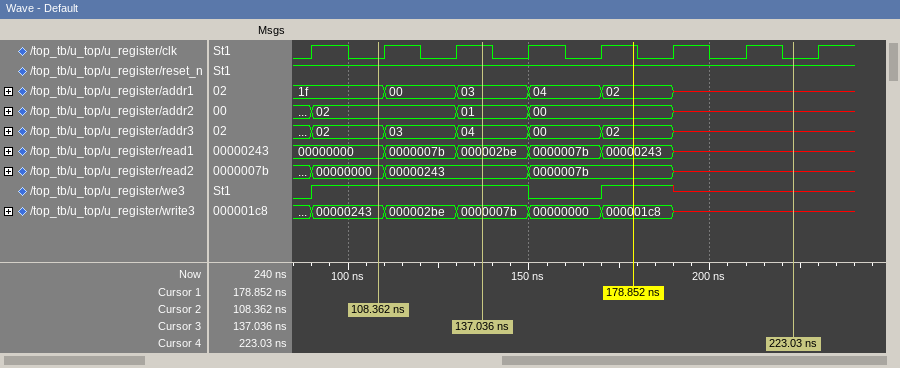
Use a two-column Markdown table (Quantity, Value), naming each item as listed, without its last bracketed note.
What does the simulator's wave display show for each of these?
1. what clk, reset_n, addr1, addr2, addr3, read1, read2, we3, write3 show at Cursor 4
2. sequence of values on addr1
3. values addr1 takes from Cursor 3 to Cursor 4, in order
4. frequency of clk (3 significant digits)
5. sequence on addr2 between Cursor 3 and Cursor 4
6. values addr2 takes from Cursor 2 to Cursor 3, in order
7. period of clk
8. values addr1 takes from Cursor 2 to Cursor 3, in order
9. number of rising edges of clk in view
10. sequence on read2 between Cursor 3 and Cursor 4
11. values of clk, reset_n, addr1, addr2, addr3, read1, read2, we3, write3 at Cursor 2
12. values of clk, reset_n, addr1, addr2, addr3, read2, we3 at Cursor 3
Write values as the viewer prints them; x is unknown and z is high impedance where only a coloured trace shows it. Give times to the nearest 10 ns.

| Quantity | Value |
|---|---|
| what clk, reset_n, addr1, addr2, addr3, read1, read2, we3, write3 show at Cursor 4 | clk=0, reset_n=1, addr1=x, addr2=x, addr3=x, read1=x, read2=x, we3=x, write3=x |
| sequence of values on addr1 | 1f, 00, 03, 04, 02, x |
| values addr1 takes from Cursor 3 to Cursor 4, in order | 03, 04, 02, x |
| frequency of clk | 50.0 MHz |
| sequence on addr2 between Cursor 3 and Cursor 4 | 01, 00, x |
| values addr2 takes from Cursor 2 to Cursor 3, in order | 02, 01 |
| period of clk | 20 ns |
| values addr1 takes from Cursor 2 to Cursor 3, in order | 1f, 00, 03 |
| number of rising edges of clk in view | 8 |
| sequence on read2 between Cursor 3 and Cursor 4 | 00000243, 0000007b, x |
| values of clk, reset_n, addr1, addr2, addr3, read1, read2, we3, write3 at Cursor 2 | clk=0, reset_n=1, addr1=1f, addr2=02, addr3=02, read1=00000000, read2=00000000, we3=1, write3=00000243 |
| values of clk, reset_n, addr1, addr2, addr3, read2, we3 at Cursor 3 | clk=1, reset_n=1, addr1=03, addr2=01, addr3=04, read2=00000243, we3=1 |
